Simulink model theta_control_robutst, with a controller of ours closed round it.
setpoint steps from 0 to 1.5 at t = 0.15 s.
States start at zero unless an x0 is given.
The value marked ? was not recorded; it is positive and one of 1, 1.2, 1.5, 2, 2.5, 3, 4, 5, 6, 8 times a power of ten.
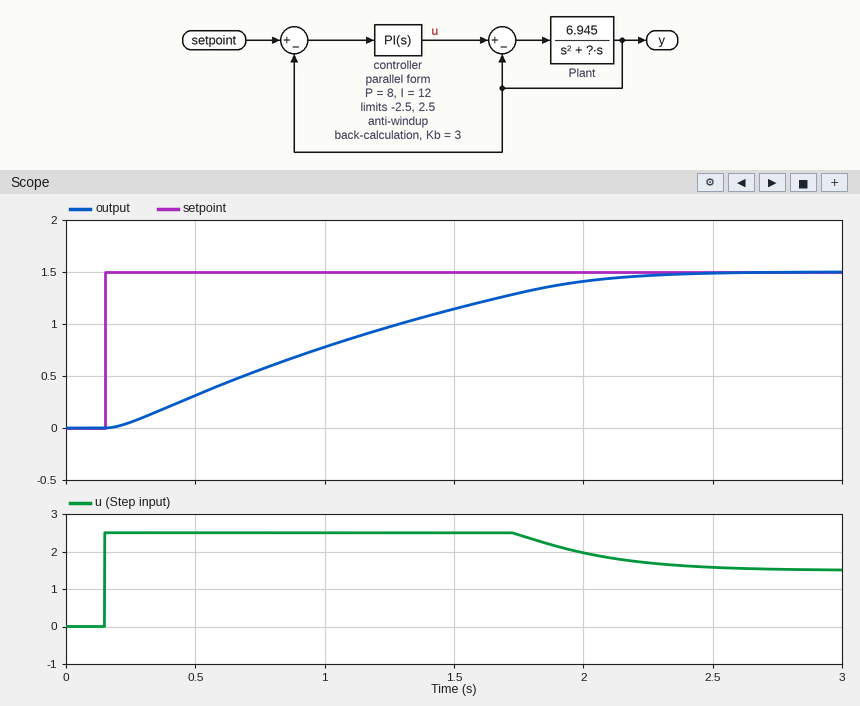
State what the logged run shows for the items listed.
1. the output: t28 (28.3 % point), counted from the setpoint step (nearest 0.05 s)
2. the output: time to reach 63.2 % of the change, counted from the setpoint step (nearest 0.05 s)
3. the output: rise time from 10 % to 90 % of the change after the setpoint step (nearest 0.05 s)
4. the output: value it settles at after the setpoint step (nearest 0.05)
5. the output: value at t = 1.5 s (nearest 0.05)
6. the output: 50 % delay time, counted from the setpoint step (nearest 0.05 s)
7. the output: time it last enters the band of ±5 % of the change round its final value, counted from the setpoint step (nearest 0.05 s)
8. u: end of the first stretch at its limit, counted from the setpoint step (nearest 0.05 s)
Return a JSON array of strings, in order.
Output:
["0.45 s", "1.05 s", "1.50 s", "1.50", "1.15", "0.80 s", "1.90 s", "1.60 s"]
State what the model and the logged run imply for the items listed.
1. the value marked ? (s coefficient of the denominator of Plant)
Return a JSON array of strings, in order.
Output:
["15"]
